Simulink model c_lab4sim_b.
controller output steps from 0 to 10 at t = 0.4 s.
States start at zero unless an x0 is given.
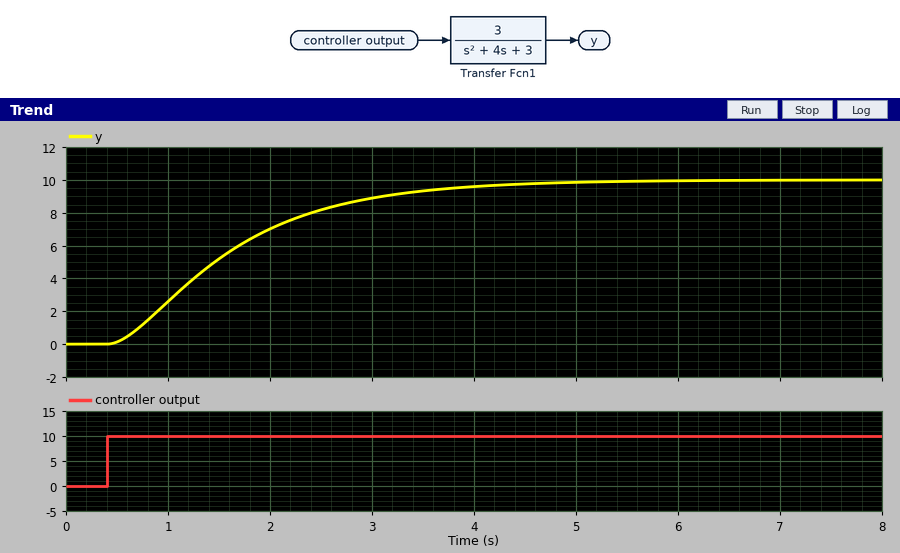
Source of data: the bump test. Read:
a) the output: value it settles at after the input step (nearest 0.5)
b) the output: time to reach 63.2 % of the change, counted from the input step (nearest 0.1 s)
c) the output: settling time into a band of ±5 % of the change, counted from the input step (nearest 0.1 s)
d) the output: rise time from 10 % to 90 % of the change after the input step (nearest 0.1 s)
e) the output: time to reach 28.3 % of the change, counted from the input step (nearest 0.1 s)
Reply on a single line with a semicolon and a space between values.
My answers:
10.0; 1.4 s; 3.4 s; 2.4 s; 0.6 s
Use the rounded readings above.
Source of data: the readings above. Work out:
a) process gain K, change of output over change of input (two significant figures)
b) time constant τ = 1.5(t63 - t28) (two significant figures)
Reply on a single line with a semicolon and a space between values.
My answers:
1.0; 1.2 s
